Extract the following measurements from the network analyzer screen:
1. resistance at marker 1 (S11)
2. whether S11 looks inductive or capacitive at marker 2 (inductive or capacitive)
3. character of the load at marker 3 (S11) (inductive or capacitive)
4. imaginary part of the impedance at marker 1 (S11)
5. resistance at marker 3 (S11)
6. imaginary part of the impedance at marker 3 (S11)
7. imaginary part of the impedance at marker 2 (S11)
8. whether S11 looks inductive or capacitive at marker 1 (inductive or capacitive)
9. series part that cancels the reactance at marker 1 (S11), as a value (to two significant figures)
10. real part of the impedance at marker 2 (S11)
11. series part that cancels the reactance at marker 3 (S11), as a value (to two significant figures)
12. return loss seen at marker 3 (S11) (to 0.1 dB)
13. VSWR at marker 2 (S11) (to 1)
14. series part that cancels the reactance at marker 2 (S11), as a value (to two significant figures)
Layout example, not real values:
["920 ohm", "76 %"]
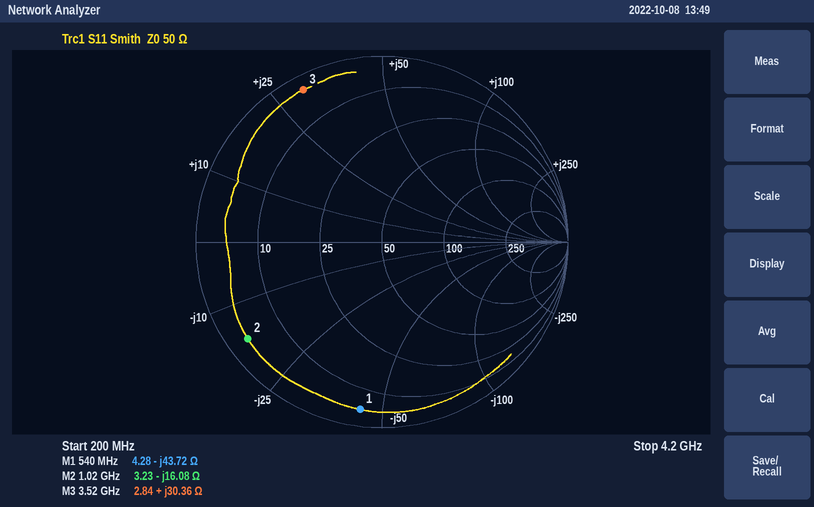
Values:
["4.28 Ω", "capacitive", "inductive", "-43.72 Ω", "2.84 Ω", "+30.36 Ω", "-16.08 Ω", "capacitive", "13 nH", "3.23 Ω", "1.5 pF", "0.7 dB", "17", "2.5 nH"]
